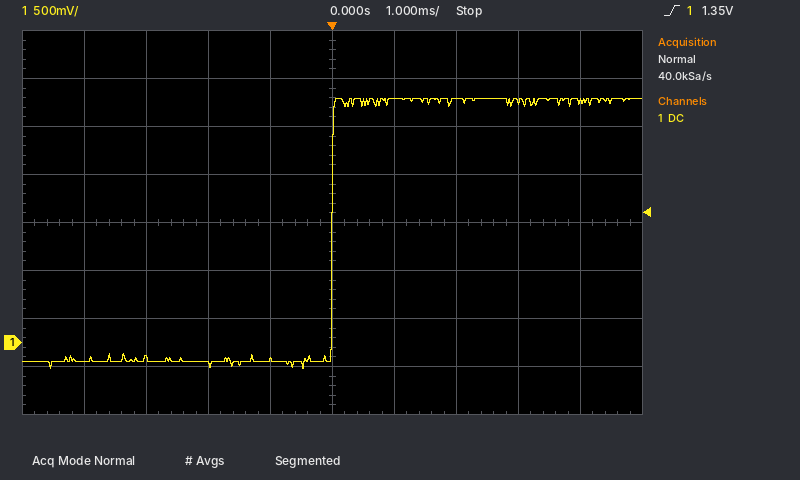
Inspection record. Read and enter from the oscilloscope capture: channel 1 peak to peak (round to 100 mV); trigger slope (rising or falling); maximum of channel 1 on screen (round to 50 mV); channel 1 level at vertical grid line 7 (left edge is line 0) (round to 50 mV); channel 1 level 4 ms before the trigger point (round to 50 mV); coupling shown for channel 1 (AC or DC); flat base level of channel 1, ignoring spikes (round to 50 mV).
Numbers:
2.80 V
rising
2.55 V
2.55 V
-200 mV
DC
-200 mV
